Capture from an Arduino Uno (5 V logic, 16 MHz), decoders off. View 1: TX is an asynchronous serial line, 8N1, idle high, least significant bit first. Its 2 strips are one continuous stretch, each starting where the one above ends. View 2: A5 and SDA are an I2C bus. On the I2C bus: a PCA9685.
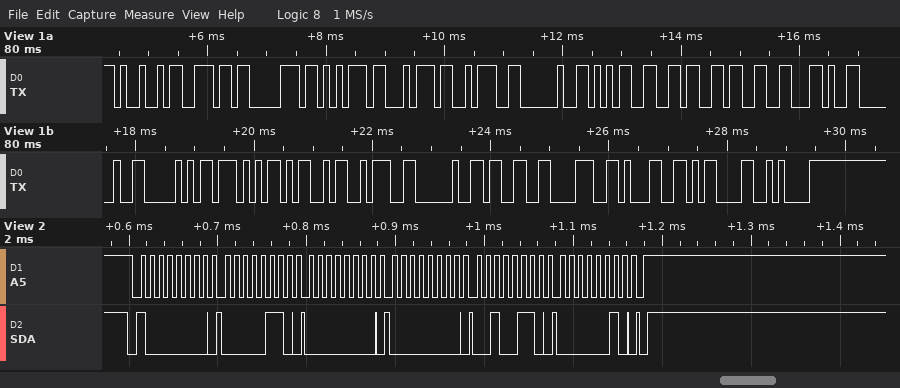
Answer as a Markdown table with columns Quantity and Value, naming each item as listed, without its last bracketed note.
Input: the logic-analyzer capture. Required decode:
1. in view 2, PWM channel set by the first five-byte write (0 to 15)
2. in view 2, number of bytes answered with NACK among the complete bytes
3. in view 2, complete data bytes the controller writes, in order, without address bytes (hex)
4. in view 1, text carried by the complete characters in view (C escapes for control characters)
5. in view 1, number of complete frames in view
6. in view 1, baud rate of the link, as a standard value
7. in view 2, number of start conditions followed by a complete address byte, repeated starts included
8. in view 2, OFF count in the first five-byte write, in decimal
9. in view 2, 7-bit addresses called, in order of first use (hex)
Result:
| Quantity | Value |
|---|---|
| in view 2, PWM channel set by the first five-byte write | 0 |
| in view 2, number of bytes answered with NACK among the complete bytes | 0 |
| in view 2, complete data bytes the controller writes, in order, without address bytes | 06 00 00 26 02 |
| in view 1, text carried by the complete characters in view | "Input: 563, PWM: 381\r\n" |
| in view 1, number of complete frames in view | 22 |
| in view 1, baud rate of the link, as a standard value | 9600 baud |
| in view 2, number of start conditions followed by a complete address byte, repeated starts included | 1 |
| in view 2, OFF count in the first five-byte write, in decimal | 550 |
| in view 2, 7-bit addresses called, in order of first use | 0x40 |
